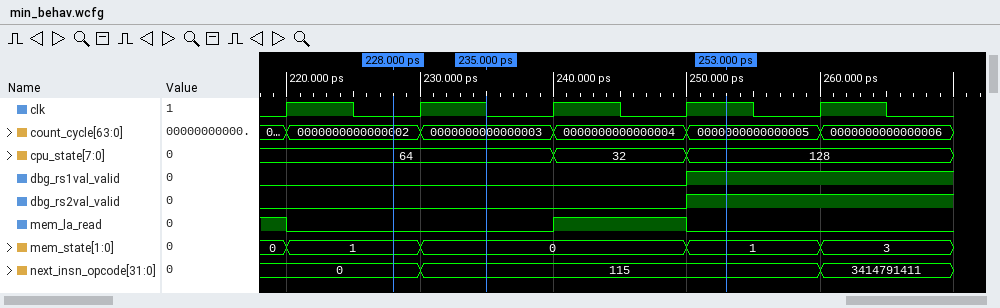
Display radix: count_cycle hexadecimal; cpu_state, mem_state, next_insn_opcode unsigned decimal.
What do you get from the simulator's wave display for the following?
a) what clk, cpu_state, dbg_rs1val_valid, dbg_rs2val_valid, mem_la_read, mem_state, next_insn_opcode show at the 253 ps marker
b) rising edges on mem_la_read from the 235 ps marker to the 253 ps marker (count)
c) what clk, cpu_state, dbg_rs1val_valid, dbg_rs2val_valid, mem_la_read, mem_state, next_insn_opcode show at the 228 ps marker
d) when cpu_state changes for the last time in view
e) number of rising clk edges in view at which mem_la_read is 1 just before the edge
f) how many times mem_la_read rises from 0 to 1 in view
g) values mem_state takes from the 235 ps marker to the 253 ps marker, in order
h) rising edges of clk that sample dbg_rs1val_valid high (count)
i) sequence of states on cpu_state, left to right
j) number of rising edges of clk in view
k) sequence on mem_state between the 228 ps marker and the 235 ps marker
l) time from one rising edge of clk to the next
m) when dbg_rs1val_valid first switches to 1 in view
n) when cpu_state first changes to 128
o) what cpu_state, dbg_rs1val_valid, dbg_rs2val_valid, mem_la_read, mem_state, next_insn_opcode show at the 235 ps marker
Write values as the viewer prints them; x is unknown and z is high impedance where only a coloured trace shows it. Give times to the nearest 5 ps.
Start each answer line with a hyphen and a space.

- clk=1, cpu_state=128, dbg_rs1val_valid=1, dbg_rs2val_valid=1, mem_la_read=0, mem_state=1, next_insn_opcode=115
- 1
- clk=0, cpu_state=64, dbg_rs1val_valid=0, dbg_rs2val_valid=0, mem_la_read=0, mem_state=1, next_insn_opcode=0
- 250 ps
- 2
- 1
- 0, 1
- 1
- 64, 32, 128
- 5
- 1, 0
- 10 ps
- 250 ps
- 250 ps
- cpu_state=64, dbg_rs1val_valid=0, dbg_rs2val_valid=0, mem_la_read=0, mem_state=0, next_insn_opcode=115
